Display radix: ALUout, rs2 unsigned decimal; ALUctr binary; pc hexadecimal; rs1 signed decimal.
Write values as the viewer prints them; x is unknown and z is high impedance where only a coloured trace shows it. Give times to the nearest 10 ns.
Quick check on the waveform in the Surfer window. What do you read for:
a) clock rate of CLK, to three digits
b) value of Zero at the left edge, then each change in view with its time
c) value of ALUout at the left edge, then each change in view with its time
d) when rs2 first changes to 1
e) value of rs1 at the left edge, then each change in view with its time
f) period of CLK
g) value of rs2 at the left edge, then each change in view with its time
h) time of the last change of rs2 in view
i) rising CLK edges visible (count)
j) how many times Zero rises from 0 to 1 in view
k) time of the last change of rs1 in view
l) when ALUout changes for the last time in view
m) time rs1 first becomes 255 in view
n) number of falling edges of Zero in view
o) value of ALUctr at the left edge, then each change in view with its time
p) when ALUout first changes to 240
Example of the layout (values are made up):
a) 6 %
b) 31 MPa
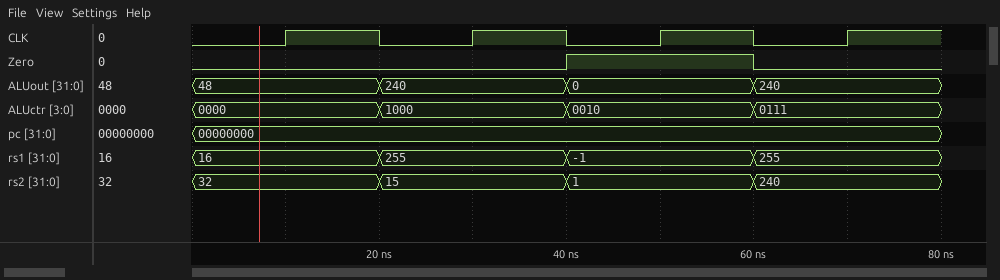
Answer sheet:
a) 50.0 MHz
b) 0, 1 at 40 ns, 0 at 60 ns
c) 48, 240 at 20 ns, 0 at 40 ns, 240 at 60 ns
d) 40 ns
e) 16, 255 at 20 ns, -1 at 40 ns, 255 at 60 ns
f) 20 ns
g) 32, 15 at 20 ns, 1 at 40 ns, 240 at 60 ns
h) 60 ns
i) 4
j) 1
k) 60 ns
l) 60 ns
m) 20 ns
n) 1
o) 0000, 1000 at 20 ns, 0010 at 40 ns, 0111 at 60 ns
p) 20 ns
